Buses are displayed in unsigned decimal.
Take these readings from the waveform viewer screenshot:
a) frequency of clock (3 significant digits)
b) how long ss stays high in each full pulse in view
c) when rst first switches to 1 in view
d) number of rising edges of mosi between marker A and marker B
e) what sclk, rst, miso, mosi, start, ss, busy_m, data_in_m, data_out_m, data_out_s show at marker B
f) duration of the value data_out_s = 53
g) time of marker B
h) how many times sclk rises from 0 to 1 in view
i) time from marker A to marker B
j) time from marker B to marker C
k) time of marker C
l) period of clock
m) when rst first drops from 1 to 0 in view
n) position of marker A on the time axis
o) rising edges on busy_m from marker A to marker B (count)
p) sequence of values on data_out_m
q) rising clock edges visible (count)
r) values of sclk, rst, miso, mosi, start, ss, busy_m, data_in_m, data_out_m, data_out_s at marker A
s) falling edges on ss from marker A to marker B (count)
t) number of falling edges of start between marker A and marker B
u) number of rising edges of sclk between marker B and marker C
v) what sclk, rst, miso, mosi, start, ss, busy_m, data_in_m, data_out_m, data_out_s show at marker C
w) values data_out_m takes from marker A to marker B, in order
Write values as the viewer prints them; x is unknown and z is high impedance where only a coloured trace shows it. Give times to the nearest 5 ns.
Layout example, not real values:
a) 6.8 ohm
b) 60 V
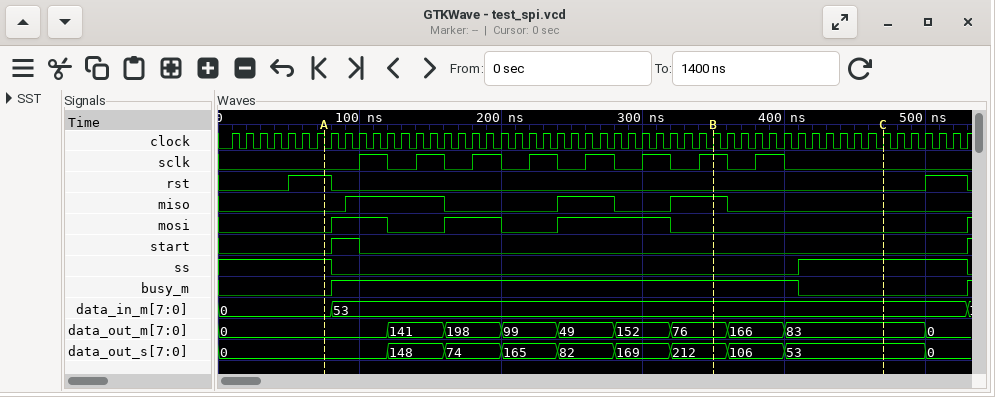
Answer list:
a) 100 MHz
b) 120 ns
c) 50 ns
d) 3
e) sclk=1, rst=0, miso=1, mosi=0, start=0, ss=0, busy_m=1, data_in_m=53, data_out_m=76, data_out_s=212
f) 100 ns
g) 350 ns
h) 8
i) 275 ns
j) 120 ns
k) 470 ns
l) 10 ns
m) 80 ns
n) 75 ns
o) 1
p) 0, 141, 198, 99, 49, 152, 76, 166, 83, 0
q) 53
r) sclk=0, rst=1, miso=0, mosi=0, start=0, ss=1, busy_m=0, data_in_m=0, data_out_m=0, data_out_s=0
s) 1
t) 1
u) 1
v) sclk=0, rst=0, miso=0, mosi=0, start=0, ss=1, busy_m=0, data_in_m=53, data_out_m=83, data_out_s=53
w) 0, 141, 198, 99, 49, 152, 76
